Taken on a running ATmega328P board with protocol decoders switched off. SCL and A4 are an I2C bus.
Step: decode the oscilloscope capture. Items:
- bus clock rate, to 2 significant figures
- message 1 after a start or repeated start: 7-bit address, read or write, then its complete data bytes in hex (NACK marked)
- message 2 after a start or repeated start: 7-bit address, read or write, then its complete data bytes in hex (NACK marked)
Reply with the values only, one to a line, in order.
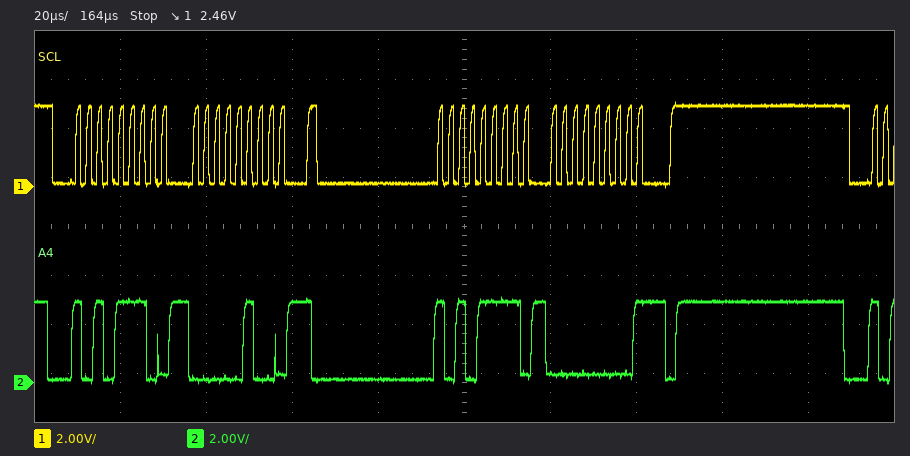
400 kHz
0x57 write: 04
0x57 read: 00 NACK
